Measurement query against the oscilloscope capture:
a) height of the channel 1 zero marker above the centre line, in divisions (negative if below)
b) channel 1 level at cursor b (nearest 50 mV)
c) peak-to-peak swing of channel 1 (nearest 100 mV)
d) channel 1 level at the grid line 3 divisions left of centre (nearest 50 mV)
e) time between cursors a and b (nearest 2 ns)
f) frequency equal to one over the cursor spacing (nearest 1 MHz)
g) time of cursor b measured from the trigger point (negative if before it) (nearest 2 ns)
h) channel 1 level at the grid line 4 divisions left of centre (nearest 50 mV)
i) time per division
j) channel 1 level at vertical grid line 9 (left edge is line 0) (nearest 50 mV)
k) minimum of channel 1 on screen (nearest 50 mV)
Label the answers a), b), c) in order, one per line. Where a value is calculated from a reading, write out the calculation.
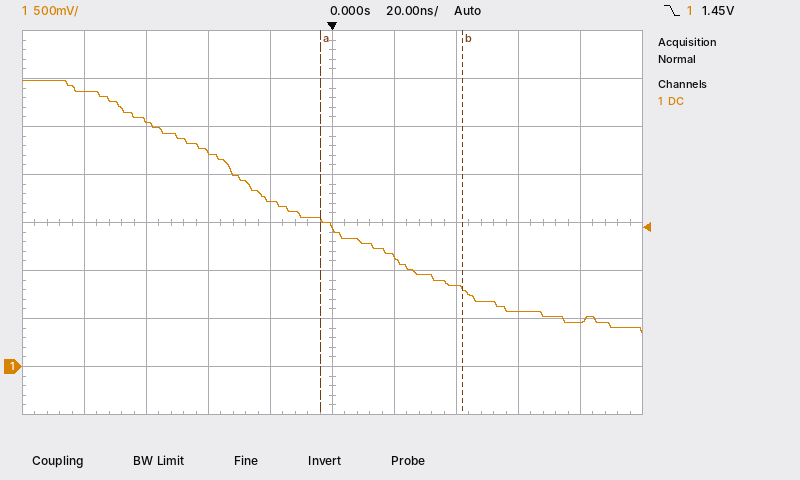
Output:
a) -3.0 div
b) 800 mV
c) 2.60 V
d) 2.55 V
e) 46 ns
f) 1 / 46 ns ≈ 22 MHz
g) +42 ns
h) 2.85 V
i) 20 ns
j) 450 mV
k) 350 mV
